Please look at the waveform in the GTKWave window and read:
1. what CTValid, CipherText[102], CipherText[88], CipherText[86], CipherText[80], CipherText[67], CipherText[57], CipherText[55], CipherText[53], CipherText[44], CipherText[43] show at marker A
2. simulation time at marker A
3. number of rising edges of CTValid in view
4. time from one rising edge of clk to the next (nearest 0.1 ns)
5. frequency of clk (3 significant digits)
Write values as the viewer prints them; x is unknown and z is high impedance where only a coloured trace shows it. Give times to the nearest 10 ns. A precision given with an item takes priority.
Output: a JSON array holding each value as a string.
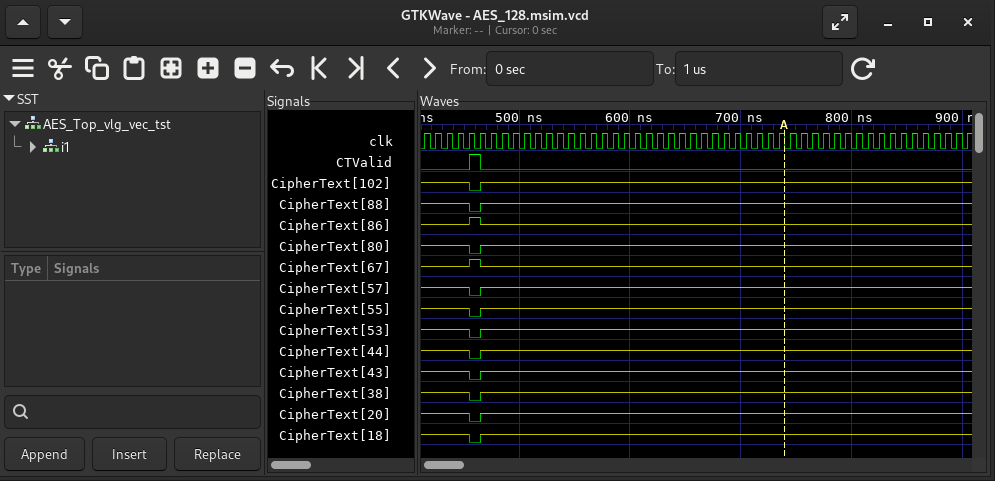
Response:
["CTValid=0, CipherText[102]=z, CipherText[88]=z, CipherText[86]=z, CipherText[80]=z, CipherText[67]=z, CipherText[57]=z, CipherText[55]=z, CipherText[53]=z, CipherText[44]=z, CipherText[43]=z", "740 ns", "1", "10 ns", "100 MHz"]
